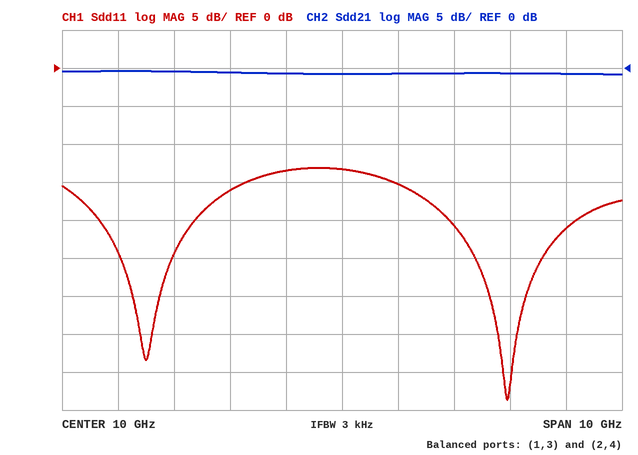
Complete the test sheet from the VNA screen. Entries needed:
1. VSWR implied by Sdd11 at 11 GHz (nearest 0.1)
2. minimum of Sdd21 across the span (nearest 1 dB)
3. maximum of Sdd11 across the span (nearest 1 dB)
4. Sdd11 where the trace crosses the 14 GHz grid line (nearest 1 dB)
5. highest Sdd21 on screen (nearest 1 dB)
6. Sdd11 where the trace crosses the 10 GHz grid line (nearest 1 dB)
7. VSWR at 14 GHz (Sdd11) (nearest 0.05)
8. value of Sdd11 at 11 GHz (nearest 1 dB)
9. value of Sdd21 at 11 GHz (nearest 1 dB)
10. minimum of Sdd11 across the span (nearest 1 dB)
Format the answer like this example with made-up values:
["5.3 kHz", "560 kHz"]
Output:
["1.4", "-1 dB", "-13 dB", "-21 dB", "0 dB", "-13 dB", "1.20", "-15 dB", "-1 dB", "-44 dB"]
